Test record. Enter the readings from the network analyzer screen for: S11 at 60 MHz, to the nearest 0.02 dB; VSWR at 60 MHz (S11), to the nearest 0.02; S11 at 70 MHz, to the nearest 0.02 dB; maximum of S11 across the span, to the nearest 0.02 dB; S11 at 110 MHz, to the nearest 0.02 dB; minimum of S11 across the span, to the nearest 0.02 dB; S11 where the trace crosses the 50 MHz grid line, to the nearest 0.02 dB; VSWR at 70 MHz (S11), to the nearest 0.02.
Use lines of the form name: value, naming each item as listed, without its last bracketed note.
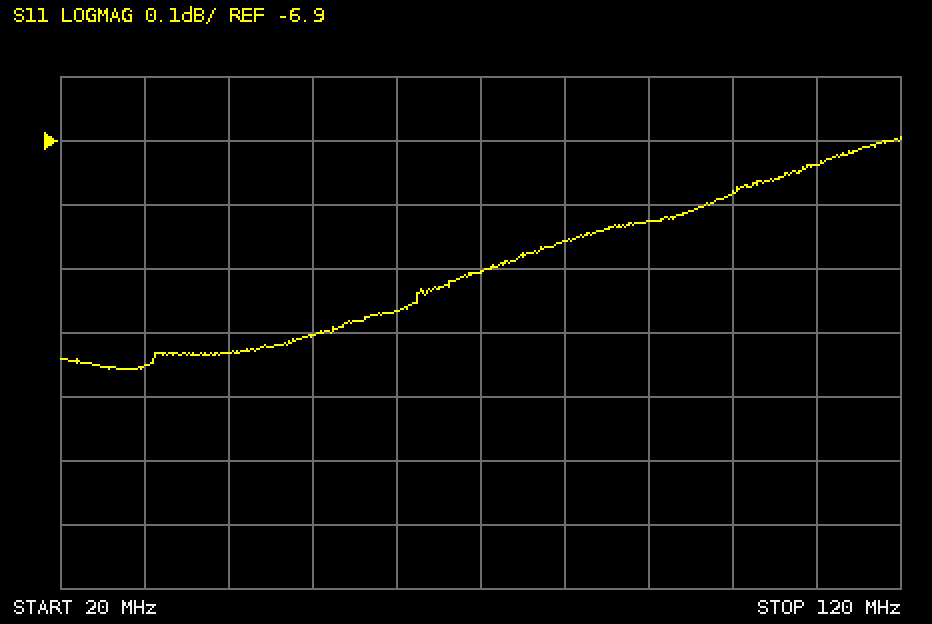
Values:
S11 at 60 MHz, to the nearest 0.02 dB: -7.16 dB
VSWR at 60 MHz (S11), to the nearest 0.02: 2.56
S11 at 70 MHz, to the nearest 0.02 dB: -7.10 dB
maximum of S11 across the span, to the nearest 0.02 dB: -6.90 dB
S11 at 110 MHz, to the nearest 0.02 dB: -6.94 dB
minimum of S11 across the span, to the nearest 0.02 dB: -7.26 dB
S11 where the trace crosses the 50 MHz grid line, to the nearest 0.02 dB: -7.20 dB
VSWR at 70 MHz (S11), to the nearest 0.02: 2.58
